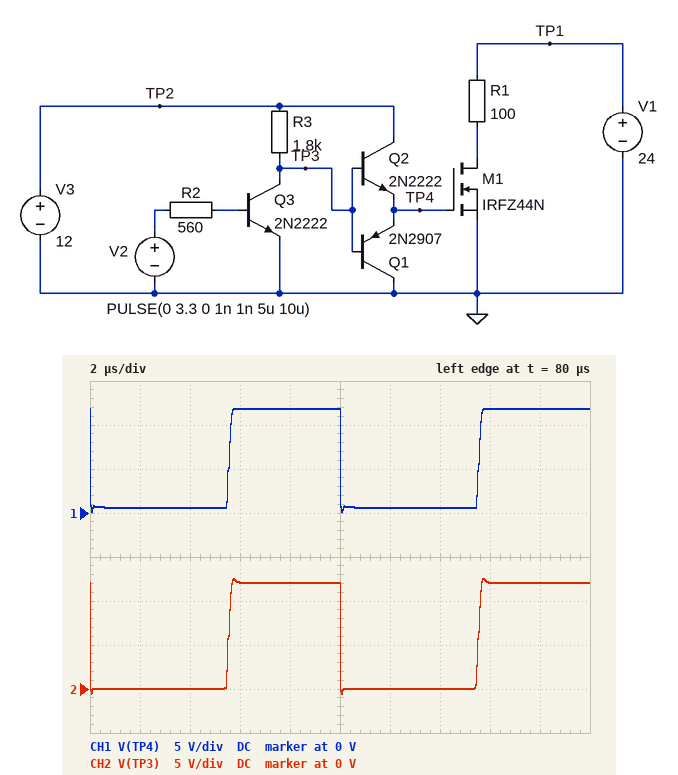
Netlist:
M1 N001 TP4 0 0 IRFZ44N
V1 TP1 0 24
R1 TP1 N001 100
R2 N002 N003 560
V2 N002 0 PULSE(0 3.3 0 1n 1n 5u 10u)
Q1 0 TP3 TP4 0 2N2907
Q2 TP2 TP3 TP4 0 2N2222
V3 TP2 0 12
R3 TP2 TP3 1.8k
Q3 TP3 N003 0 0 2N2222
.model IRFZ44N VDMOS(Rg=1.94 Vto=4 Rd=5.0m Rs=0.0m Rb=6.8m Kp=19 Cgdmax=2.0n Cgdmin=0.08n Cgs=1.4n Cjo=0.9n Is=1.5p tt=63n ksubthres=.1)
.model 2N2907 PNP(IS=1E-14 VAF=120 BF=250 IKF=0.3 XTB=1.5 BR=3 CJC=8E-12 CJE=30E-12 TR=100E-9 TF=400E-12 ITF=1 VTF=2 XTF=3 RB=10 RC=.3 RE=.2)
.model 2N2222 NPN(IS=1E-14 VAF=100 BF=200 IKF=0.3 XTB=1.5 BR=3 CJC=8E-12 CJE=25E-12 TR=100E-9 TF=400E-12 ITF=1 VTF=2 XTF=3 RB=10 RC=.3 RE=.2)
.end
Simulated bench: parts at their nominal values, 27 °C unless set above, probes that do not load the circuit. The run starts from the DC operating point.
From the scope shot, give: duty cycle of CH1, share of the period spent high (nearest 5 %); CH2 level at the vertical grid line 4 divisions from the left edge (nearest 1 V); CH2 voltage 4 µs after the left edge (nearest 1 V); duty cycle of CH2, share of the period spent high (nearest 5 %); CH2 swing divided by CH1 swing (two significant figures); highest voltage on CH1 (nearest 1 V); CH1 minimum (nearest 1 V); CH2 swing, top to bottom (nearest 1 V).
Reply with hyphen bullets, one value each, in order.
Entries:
- 45 %
- 12 V
- 0 V
- 45 %
- 1.1
- 12 V
- 0 V
- 13 V
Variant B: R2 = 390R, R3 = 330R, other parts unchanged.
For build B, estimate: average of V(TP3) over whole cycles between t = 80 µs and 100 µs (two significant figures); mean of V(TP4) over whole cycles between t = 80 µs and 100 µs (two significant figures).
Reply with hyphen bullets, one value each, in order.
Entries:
- 5.5 V
- 5.8 V
